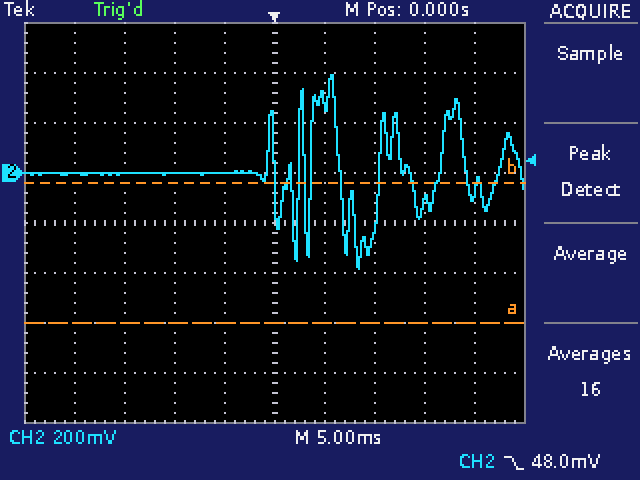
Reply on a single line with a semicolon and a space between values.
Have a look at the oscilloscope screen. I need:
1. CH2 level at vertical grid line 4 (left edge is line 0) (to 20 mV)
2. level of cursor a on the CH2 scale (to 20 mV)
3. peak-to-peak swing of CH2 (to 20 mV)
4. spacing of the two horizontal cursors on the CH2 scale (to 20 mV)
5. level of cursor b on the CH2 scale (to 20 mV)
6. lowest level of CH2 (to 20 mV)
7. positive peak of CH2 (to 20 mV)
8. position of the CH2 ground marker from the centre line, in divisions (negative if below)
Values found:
0 mV; -600 mV; 780 mV; 560 mV; -40 mV; -380 mV; 400 mV; +1.0 div
